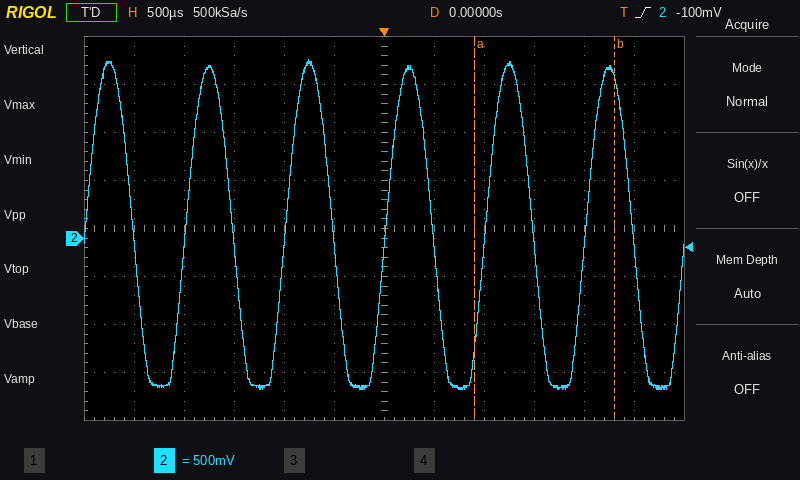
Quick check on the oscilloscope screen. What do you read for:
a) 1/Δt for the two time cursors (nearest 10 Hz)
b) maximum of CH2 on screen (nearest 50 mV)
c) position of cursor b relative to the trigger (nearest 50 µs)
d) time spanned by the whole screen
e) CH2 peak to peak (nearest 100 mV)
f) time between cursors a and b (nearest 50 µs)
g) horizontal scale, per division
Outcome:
710 Hz
1.85 V
+2.30 ms
6 ms
3.40 V
1.40 ms
500 µs
